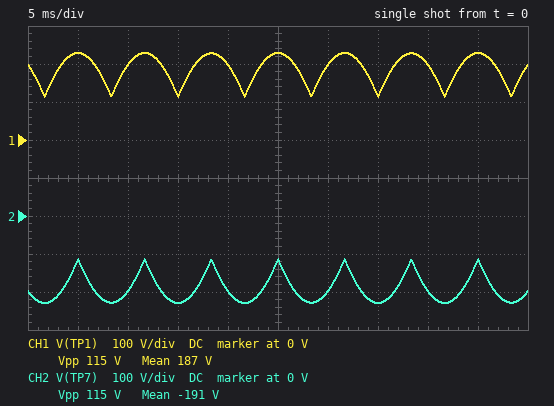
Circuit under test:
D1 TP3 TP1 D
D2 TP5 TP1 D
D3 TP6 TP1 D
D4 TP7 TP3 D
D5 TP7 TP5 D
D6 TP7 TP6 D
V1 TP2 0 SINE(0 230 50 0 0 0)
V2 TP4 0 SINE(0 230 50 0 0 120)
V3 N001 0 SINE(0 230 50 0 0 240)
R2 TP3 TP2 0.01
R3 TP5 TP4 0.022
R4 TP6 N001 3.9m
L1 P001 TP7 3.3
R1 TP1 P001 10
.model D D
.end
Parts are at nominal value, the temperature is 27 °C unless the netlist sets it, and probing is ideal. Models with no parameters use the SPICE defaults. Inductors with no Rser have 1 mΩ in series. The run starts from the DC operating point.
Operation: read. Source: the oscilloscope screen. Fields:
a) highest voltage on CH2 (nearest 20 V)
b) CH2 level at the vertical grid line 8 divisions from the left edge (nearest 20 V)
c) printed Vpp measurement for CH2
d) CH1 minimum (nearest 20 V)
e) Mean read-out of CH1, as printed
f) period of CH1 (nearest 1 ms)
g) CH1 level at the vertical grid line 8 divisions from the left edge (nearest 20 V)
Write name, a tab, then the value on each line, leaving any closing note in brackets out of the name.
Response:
highest voltage on CH2	-120 V
CH2 level at the vertical grid line 8 divisions from the left edge	-200 V
printed Vpp measurement for CH2	115 V
CH1 minimum	120 V
Mean read-out of CH1, as printed	187 V
period of CH1	7 ms
CH1 level at the vertical grid line 8 divisions from the left edge	200 V
